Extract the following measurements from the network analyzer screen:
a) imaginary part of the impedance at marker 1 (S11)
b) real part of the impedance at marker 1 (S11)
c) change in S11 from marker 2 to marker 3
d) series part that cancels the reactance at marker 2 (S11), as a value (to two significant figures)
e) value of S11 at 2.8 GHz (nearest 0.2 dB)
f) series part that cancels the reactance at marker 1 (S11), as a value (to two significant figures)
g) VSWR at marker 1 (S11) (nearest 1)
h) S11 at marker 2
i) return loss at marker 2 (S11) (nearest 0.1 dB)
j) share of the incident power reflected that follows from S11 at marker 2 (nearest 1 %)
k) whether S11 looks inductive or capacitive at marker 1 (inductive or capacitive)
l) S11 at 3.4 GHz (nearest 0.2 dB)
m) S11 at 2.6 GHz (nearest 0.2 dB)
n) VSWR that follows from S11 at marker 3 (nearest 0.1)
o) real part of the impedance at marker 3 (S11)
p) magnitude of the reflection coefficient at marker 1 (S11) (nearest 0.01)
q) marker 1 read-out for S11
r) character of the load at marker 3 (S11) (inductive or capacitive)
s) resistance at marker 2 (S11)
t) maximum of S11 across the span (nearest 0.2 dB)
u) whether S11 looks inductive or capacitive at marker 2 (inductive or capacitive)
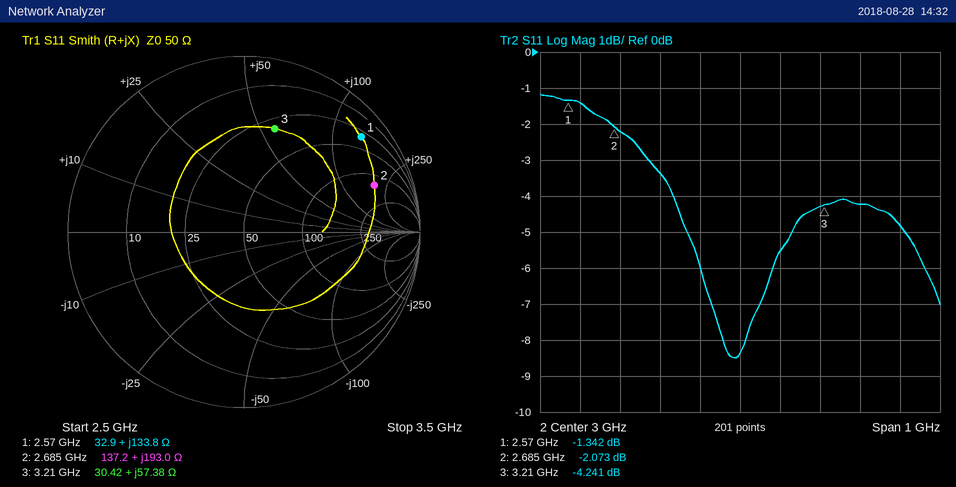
+133.8 Ω
32.9 Ω
-2.168 dB
310 fF
-3.4 dB
460 fF
13
-2.073 dB
2.1 dB
62 %
inductive
-4.8 dB
-1.4 dB
4.2
30.42 Ω
0.86
-1.342 dB
inductive
137.2 Ω
-1.2 dB
inductive
